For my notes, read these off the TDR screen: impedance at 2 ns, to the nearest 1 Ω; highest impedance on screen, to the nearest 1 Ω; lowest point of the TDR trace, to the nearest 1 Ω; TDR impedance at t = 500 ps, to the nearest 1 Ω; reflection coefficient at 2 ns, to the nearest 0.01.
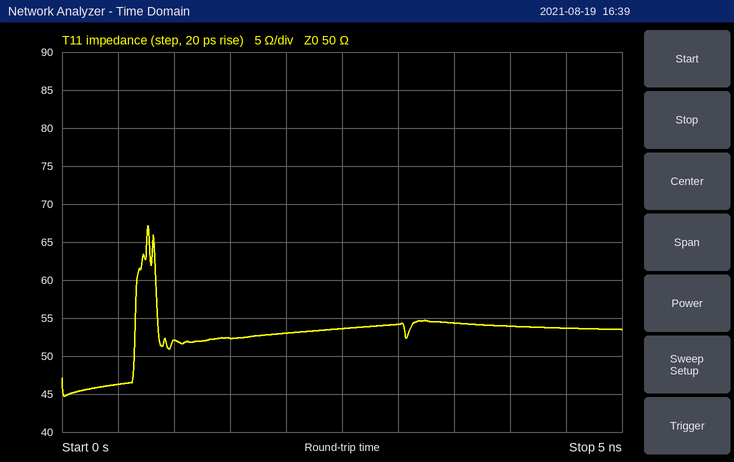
53 Ω
67 Ω
45 Ω
46 Ω
+0.03
